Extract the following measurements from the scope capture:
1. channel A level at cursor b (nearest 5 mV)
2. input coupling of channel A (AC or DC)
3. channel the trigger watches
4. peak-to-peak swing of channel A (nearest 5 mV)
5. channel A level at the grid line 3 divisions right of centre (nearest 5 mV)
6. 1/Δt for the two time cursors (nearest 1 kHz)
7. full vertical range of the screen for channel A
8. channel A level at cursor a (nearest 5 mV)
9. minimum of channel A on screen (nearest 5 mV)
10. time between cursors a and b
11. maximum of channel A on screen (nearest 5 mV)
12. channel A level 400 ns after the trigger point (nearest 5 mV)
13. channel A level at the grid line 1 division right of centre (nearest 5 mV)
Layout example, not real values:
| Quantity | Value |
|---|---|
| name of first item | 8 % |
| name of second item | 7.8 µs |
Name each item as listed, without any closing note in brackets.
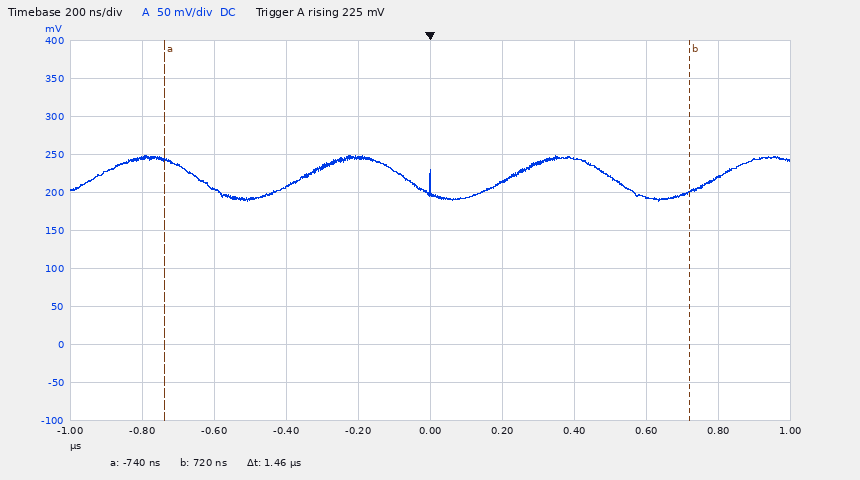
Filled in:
| Quantity | Value |
|---|---|
| channel A level at cursor b | 200 mV |
| input coupling of channel A | DC |
| channel the trigger watches | channel A |
| peak-to-peak swing of channel A | 60 mV |
| channel A level at the grid line 3 divisions right of centre | 195 mV |
| 1/Δt for the two time cursors | 685 kHz |
| full vertical range of the screen for channel A | 500 mV |
| channel A level at cursor a | 245 mV |
| minimum of channel A on screen | 190 mV |
| time between cursors a and b | 1.46 µs |
| maximum of channel A on screen | 250 mV |
| channel A level 400 ns after the trigger point | 245 mV |
| channel A level at the grid line 1 division right of centre | 215 mV |
